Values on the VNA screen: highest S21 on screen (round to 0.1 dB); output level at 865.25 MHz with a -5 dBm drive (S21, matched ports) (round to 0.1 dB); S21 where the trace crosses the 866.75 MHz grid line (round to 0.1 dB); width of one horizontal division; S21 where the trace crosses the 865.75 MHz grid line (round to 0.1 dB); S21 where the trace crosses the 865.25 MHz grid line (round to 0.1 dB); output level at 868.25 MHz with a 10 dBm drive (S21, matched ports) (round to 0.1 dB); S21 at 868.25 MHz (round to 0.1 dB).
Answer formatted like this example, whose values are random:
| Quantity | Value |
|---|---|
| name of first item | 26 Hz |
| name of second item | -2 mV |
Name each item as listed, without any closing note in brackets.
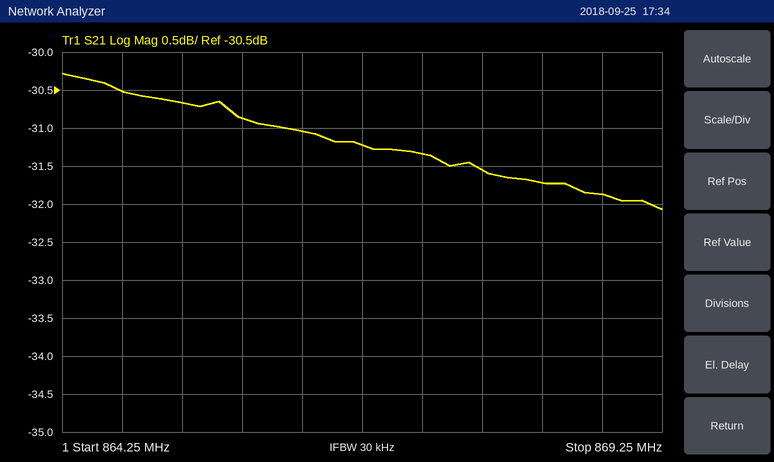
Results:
| Quantity | Value |
|---|---|
| highest S21 on screen | -30.3 dB |
| output level at 865.25 MHz with a -5 dBm drive (S21, matched ports) | -35.7 dBm |
| S21 where the trace crosses the 866.75 MHz grid line | -31.2 dB |
| width of one horizontal division | 500 kHz |
| S21 where the trace crosses the 865.75 MHz grid line | -30.9 dB |
| S21 where the trace crosses the 865.25 MHz grid line | -30.7 dB |
| output level at 868.25 MHz with a 10 dBm drive (S21, matched ports) | -21.7 dBm |
| S21 at 868.25 MHz | -31.7 dB |
